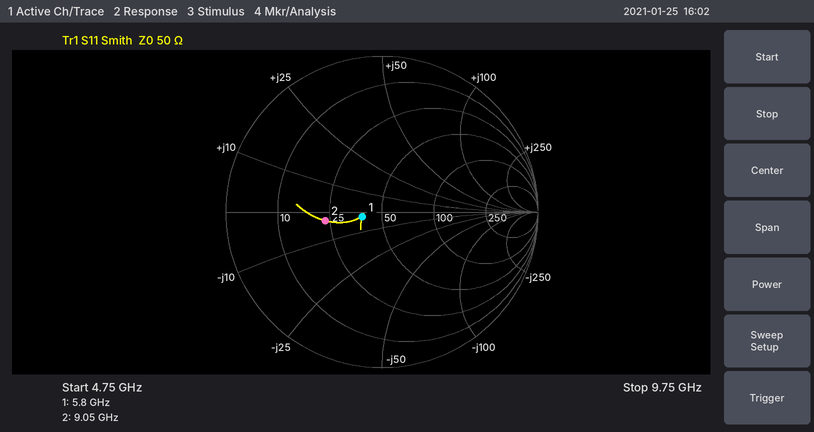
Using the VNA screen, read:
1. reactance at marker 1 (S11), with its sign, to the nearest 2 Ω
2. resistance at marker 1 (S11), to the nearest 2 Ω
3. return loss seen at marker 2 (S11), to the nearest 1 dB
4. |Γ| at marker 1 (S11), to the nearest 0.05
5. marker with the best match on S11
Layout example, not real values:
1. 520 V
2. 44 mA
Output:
1. -2 Ω
2. 38 Ω
3. 9 dB
4. 0.15
5. marker 1
